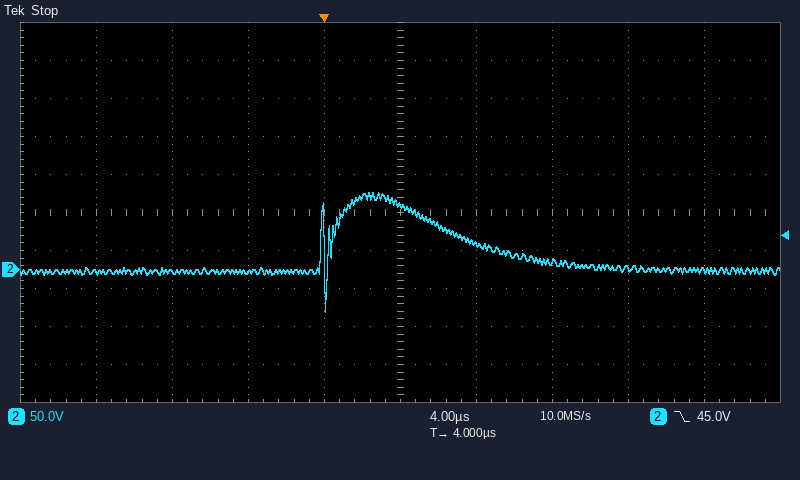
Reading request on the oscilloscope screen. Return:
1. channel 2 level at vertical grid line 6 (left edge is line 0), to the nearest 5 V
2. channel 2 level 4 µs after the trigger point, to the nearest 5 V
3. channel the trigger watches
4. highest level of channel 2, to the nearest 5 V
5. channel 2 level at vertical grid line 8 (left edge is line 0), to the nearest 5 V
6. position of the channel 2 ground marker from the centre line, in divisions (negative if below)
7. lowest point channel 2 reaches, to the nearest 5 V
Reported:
35 V
85 V
channel 2
100 V
0 V
-1.5 div
-55 V
